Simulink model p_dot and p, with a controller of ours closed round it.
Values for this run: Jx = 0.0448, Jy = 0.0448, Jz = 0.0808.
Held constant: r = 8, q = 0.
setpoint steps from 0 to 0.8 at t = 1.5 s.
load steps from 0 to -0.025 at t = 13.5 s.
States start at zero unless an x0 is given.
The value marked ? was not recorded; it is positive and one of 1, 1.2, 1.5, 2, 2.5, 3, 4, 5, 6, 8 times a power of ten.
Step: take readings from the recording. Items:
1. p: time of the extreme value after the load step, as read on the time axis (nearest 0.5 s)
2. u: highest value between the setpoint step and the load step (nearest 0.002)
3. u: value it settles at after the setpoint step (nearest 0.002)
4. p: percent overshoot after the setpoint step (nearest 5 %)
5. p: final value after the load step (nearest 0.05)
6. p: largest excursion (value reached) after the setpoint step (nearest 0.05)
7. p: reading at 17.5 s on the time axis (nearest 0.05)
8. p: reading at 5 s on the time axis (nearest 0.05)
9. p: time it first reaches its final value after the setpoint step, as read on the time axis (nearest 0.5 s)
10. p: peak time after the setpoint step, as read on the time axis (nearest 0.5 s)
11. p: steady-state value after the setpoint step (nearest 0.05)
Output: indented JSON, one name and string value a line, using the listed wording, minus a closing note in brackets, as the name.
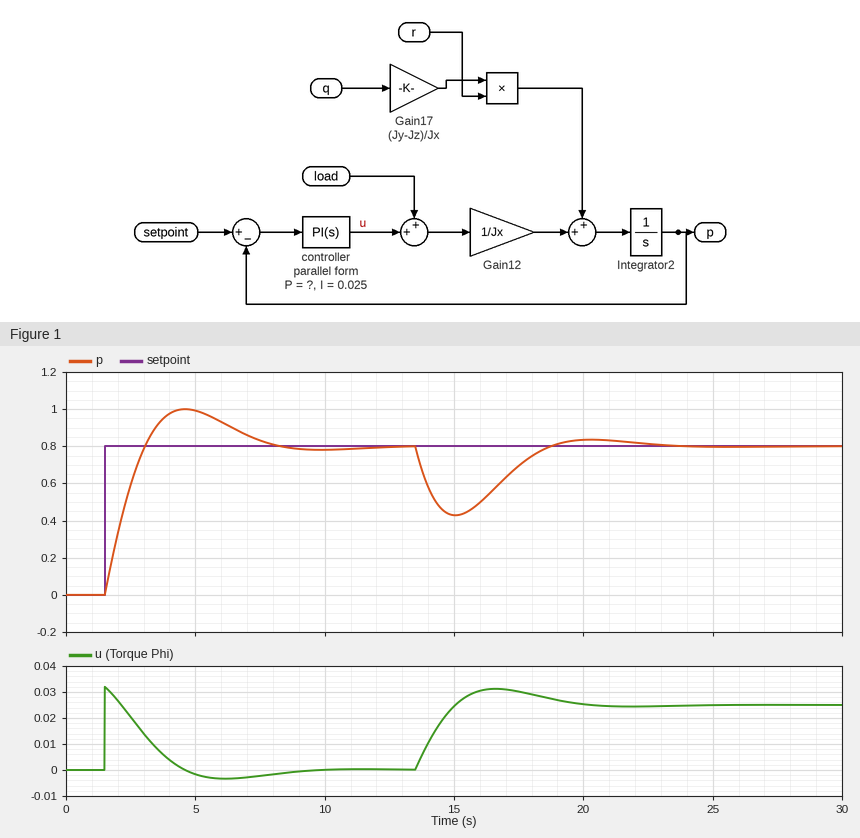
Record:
{
  "p: time of the extreme value after the load step, as read on the time axis": "15.0 s",
  "u: highest value between the setpoint step and the load step": "0.032",
  "u: value it settles at after the setpoint step": "0.000",
  "p: percent overshoot after the setpoint step": "25 %",
  "p: final value after the load step": "0.80",
  "p: largest excursion (value reached) after the setpoint step": "1.00",
  "p: reading at 17.5 s on the time axis": "0.70",
  "p: reading at 5 s on the time axis": "1.00",
  "p: time it first reaches its final value after the setpoint step, as read on the time axis": "3.0 s",
  "p: peak time after the setpoint step, as read on the time axis": "4.5 s",
  "p: steady-state value after the setpoint step": "0.80"
}
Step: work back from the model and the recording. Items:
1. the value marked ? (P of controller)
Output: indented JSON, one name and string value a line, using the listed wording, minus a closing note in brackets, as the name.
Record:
{
  "the value marked ?": "0.04"
}
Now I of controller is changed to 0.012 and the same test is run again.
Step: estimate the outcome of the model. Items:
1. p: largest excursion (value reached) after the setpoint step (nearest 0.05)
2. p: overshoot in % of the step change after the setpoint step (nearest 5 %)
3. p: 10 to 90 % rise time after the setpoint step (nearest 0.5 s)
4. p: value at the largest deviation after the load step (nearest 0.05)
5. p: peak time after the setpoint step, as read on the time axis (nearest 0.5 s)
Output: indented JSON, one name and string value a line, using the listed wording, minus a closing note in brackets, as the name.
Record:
{
  "p: largest excursion (value reached) after the setpoint step": "0.95",
  "p: overshoot in % of the step change after the setpoint step": "15 %",
  "p: 10 to 90 % rise time after the setpoint step": "1.5 s",
  "p: value at the largest deviation after the load step": "0.35",
  "p: peak time after the setpoint step, as read on the time axis": "5.5 s"
}
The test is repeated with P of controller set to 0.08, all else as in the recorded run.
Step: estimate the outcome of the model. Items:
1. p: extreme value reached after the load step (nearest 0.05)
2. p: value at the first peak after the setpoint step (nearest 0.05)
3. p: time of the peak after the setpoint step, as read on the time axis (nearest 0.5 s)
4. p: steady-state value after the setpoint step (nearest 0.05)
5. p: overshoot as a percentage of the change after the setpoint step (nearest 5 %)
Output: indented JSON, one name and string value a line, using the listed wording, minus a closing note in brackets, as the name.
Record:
{
  "p: extreme value reached after the load step": "0.55",
  "p: value at the first peak after the setpoint step": "0.90",
  "p: time of the peak after the setpoint step, as read on the time axis": "4.0 s",
  "p: steady-state value after the setpoint step": "0.80",
  "p: overshoot as a percentage of the change after the setpoint step": "10 %"
}
